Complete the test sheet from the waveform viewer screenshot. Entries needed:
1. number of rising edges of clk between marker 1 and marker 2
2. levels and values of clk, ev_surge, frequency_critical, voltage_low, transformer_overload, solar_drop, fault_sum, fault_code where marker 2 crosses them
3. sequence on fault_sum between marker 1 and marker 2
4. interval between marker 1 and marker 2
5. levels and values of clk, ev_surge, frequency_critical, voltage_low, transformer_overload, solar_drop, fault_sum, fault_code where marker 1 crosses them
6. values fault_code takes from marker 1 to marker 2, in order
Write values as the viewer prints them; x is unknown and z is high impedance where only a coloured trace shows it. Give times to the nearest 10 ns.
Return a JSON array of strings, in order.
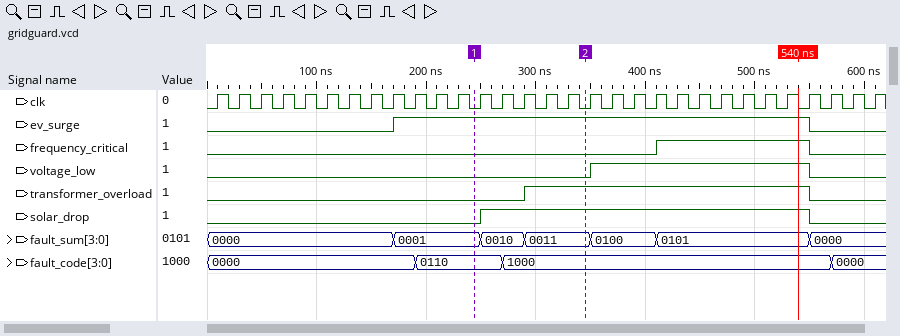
["5", "clk=0, ev_surge=1, frequency_critical=0, voltage_low=0, transformer_overload=1, solar_drop=1, fault_sum=0011, fault_code=1000", "0001, 0010, 0011", "100 ns", "clk=0, ev_surge=1, frequency_critical=0, voltage_low=0, transformer_overload=0, solar_drop=0, fault_sum=0001, fault_code=0110", "0110, 1000"]
